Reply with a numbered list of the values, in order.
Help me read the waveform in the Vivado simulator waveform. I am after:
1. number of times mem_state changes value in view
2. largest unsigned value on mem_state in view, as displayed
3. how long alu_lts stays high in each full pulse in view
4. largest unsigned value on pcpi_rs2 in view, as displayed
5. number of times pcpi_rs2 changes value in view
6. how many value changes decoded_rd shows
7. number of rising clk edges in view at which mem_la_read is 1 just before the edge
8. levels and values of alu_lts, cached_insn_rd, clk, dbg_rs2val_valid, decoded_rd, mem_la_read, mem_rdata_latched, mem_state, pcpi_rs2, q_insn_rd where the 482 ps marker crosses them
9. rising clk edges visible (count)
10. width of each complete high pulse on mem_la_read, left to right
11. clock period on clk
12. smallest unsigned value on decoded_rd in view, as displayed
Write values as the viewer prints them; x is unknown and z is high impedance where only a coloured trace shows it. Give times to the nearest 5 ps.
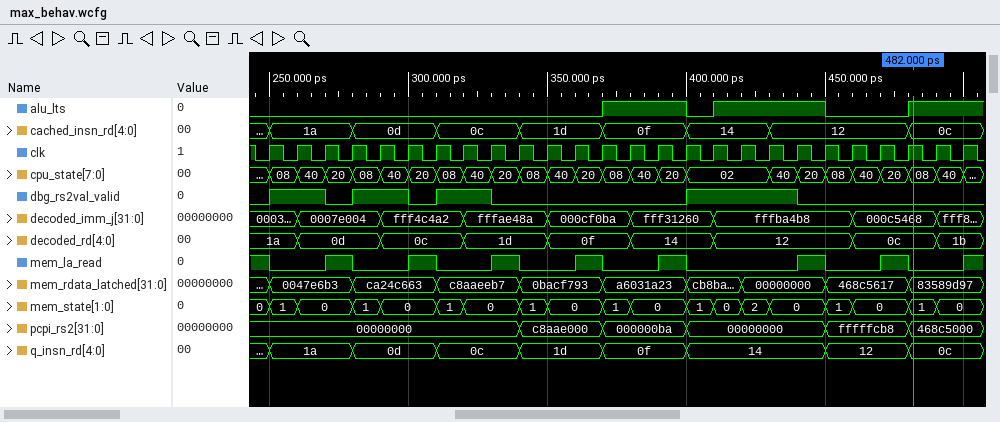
1. 18
2. 2
3. 30 ps, 40 ps
4. fffffcb8
5. 5
6. 8
7. 8
8. alu_lts=1, cached_insn_rd=0c, clk=1, dbg_rs2val_valid=0, decoded_rd=0c, mem_la_read=0, mem_rdata_latched=83589d97, mem_state=1, pcpi_rs2=468c5000, q_insn_rd=0c
9. 26
10. 10 ps, 10 ps, 10 ps, 10 ps, 10 ps, 10 ps, 10 ps
11. 10 ps
12. 0c
